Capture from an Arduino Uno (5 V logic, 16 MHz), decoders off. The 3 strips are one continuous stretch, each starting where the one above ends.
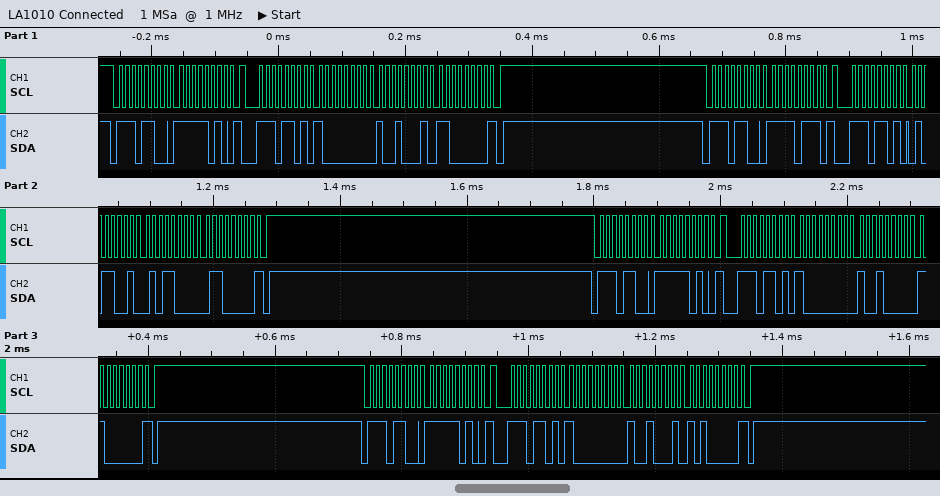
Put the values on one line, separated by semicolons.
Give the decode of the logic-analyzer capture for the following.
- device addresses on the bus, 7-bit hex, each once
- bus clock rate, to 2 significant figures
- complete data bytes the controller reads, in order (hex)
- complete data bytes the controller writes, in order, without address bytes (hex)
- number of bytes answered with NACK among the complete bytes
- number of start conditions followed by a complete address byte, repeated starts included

0x76; 100 kHz; 80 91 C0 59 58 60 80 90 C0 80 91 A0; FA F7 FA FA; 4; 8
